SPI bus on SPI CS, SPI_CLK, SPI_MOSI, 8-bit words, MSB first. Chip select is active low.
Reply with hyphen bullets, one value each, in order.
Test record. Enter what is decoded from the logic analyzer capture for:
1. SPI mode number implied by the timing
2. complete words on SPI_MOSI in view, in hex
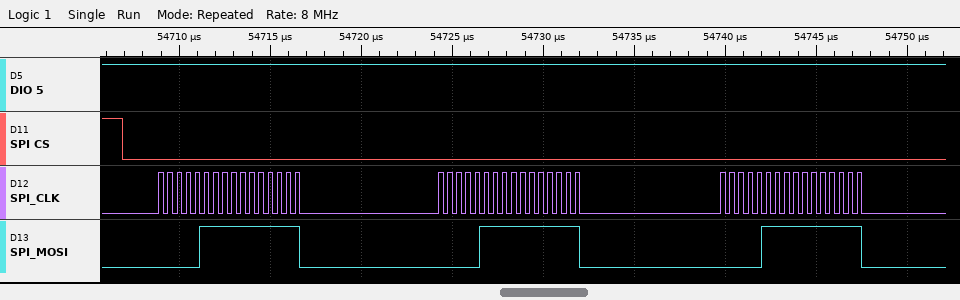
- 0
- 07, FF, 07, FF, 07, FF
